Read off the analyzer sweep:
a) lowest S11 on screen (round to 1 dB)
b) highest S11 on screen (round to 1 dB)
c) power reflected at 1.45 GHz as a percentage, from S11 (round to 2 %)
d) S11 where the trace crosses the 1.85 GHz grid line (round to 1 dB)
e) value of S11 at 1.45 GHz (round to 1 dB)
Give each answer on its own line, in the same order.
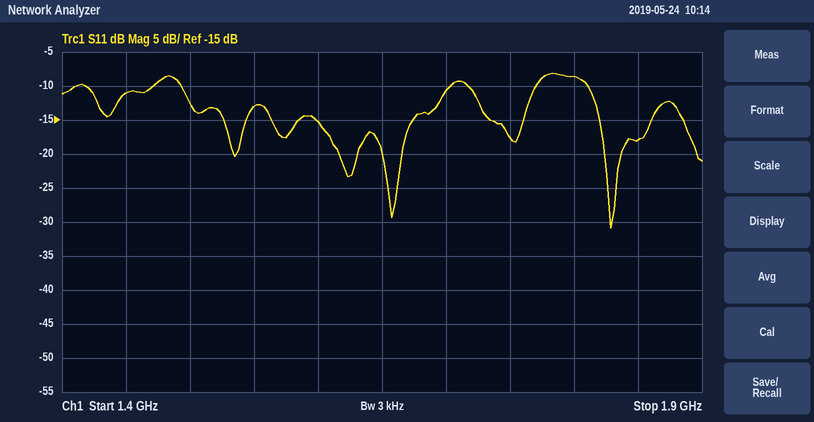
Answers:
-31 dB
-8 dB
8 %
-18 dB
-11 dB
